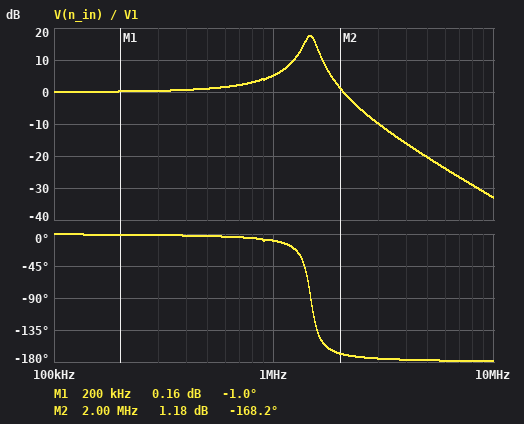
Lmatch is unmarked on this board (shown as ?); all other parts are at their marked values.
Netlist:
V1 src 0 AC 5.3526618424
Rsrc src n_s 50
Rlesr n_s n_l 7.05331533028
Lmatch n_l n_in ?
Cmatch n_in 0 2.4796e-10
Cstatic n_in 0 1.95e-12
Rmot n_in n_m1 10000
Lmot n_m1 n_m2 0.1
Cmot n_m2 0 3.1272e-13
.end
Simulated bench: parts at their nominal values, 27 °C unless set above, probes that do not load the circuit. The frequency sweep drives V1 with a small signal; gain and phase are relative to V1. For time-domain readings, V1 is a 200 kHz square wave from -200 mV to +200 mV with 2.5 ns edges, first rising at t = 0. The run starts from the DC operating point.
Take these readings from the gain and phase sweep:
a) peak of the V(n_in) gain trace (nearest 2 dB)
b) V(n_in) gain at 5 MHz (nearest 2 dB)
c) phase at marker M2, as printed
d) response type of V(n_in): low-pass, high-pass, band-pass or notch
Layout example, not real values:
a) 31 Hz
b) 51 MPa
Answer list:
a) 18 dB
b) -20 dB
c) -168.2 deg
d) low-pass
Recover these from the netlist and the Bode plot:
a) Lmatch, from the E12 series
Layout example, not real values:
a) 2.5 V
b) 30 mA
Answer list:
a) 47 µH
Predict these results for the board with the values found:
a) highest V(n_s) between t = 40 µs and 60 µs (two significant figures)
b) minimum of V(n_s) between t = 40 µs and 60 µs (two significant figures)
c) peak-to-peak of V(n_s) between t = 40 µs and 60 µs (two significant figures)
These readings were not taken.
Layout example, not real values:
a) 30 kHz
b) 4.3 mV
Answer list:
a) 240 mV
b) -240 mV
c) 480 mV
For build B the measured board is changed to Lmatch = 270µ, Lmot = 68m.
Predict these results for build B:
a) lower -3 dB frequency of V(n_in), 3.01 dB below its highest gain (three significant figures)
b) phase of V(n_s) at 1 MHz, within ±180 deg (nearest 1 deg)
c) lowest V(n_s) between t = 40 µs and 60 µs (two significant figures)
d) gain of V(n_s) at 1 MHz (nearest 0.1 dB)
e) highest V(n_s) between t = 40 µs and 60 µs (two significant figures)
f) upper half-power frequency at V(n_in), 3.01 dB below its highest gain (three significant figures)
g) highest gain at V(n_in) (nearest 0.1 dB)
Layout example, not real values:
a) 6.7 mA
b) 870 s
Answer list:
a) 595 kHz
b) 3 deg
c) -260 mV
d) 0 dB
e) 260 mV
f) 628 kHz
g) 25.2 dB
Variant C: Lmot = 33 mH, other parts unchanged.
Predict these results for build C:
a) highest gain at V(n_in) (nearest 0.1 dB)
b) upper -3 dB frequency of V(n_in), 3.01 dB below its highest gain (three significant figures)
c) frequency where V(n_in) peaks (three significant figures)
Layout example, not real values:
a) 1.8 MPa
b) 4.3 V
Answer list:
a) 17.5 dB
b) 1.53 MHz
c) 1.45 MHz
